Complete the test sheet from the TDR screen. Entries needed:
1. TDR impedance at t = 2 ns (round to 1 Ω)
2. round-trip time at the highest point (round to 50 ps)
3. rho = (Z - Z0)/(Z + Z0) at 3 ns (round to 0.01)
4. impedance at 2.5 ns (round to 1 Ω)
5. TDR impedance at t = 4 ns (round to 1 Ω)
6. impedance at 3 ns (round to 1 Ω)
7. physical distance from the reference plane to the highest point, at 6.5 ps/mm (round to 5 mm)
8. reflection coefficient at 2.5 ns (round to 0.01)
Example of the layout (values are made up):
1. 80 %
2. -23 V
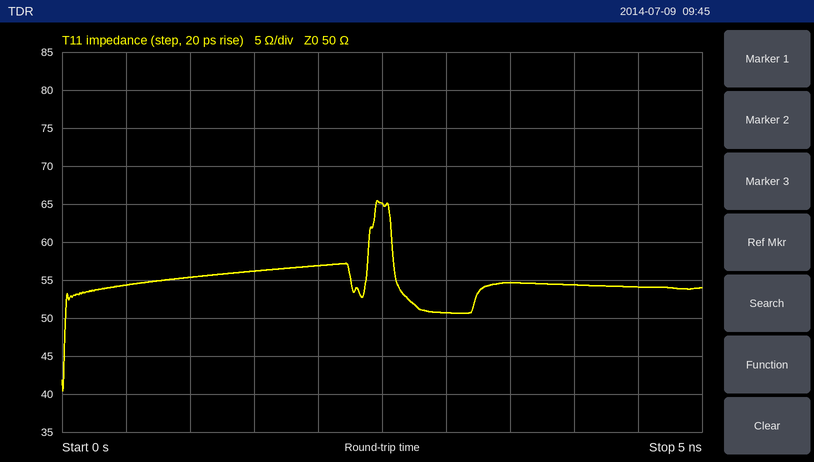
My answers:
1. 57 Ω
2. 2.45 ns
3. +0.01
4. 65 Ω
5. 54 Ω
6. 51 Ω
7. 190 mm
8. +0.13
